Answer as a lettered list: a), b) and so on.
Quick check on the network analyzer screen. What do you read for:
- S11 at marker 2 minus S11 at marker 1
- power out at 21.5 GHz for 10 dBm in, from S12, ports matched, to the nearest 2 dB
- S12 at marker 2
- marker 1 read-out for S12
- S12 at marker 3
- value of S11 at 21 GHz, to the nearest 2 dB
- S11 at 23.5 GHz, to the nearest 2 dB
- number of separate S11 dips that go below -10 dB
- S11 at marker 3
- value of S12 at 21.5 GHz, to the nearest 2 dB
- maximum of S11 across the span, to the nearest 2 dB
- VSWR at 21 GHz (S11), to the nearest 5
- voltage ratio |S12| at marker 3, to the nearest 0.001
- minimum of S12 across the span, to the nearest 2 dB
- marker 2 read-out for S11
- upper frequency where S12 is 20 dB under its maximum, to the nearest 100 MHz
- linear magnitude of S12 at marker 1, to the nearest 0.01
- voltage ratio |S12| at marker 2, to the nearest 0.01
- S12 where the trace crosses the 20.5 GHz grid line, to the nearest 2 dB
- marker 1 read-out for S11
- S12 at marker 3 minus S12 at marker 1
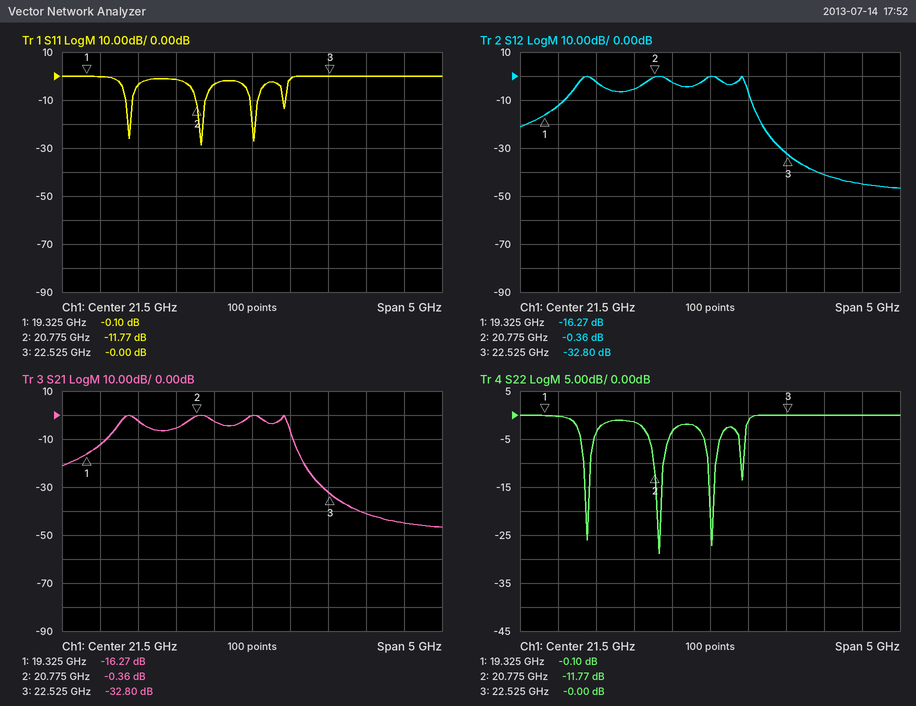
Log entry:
a) -11.67 dB
b) 10 dBm
c) -0.36 dB
d) -16.27 dB
e) -32.80 dB
f) -4 dB
g) 0 dB
h) 4
i) -0.00 dB
j) 0 dB
k) 0 dB
l) 5
m) 0.023
n) -46 dB
o) -11.77 dB
p) 22.2 GHz
q) 0.15
r) 0.96
s) -6 dB
t) -0.10 dB
u) -16.53 dB
